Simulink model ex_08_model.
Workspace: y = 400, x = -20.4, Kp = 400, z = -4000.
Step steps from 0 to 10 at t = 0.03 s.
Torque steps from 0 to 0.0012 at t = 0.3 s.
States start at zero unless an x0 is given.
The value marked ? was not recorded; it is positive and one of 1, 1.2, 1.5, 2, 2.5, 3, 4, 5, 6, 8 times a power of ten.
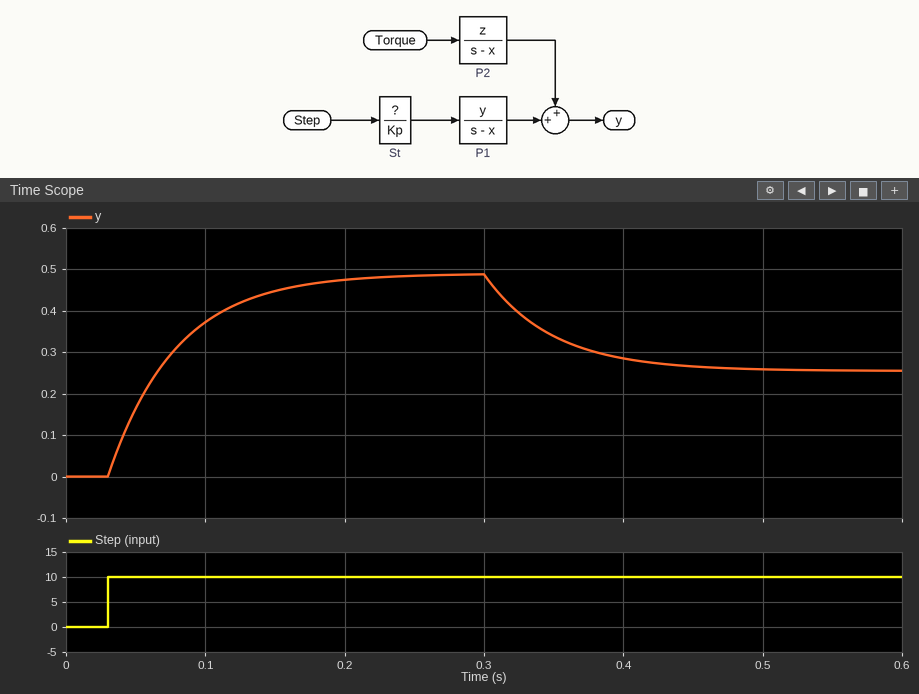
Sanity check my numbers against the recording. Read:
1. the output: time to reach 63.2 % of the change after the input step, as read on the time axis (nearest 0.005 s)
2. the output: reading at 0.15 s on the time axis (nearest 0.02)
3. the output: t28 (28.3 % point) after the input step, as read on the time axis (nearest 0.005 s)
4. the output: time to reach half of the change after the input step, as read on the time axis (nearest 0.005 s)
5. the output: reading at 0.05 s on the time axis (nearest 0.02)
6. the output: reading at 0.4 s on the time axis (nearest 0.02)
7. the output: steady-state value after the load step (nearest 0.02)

0.080 s
0.44
0.045 s
0.065 s
0.16
0.28
0.26
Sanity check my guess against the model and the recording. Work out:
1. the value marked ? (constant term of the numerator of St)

1
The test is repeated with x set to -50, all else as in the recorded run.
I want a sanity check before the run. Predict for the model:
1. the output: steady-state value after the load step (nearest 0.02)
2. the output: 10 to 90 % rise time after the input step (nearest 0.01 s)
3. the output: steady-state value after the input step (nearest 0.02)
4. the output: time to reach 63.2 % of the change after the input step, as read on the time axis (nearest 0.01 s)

0.10
0.04 s
0.20
0.05 s
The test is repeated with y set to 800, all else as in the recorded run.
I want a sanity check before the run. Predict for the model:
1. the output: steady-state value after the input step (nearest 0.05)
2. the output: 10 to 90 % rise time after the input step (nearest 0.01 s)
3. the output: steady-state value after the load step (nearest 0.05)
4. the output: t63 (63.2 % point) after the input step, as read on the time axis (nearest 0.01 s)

1.00
0.11 s
0.75
0.08 s
